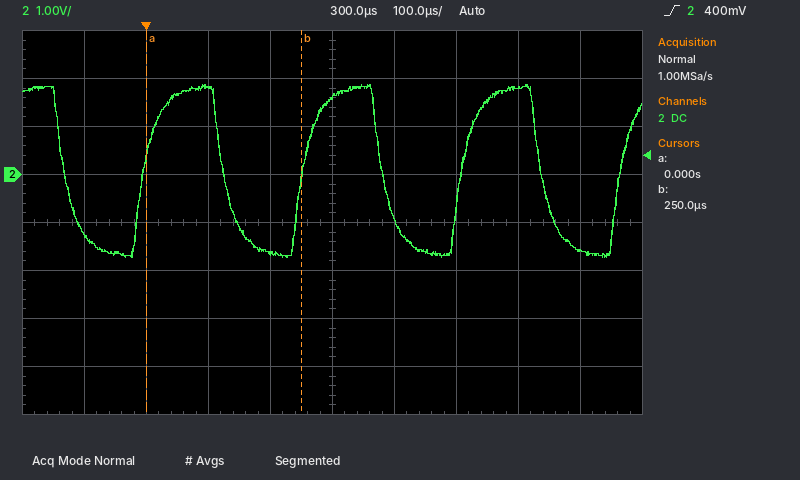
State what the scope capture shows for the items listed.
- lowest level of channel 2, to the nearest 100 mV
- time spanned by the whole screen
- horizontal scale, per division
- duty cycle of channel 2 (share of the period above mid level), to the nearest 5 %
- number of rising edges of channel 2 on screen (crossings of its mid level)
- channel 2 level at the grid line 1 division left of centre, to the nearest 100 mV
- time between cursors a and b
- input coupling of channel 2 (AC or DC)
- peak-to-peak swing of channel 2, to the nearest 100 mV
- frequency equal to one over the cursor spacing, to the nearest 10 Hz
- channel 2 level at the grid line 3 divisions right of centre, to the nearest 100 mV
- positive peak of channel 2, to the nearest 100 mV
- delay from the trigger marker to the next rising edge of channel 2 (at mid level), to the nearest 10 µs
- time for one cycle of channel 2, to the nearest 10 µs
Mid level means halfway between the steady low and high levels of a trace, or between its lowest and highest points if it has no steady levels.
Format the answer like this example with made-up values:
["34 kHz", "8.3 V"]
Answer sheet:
["-1.7 V", "1 ms", "100 µs", "50 %", "4", "-1.6 V", "250 µs", "DC", "3.6 V", "4.00 kHz", "1.8 V", "1.9 V", "250 µs", "260 µs"]
